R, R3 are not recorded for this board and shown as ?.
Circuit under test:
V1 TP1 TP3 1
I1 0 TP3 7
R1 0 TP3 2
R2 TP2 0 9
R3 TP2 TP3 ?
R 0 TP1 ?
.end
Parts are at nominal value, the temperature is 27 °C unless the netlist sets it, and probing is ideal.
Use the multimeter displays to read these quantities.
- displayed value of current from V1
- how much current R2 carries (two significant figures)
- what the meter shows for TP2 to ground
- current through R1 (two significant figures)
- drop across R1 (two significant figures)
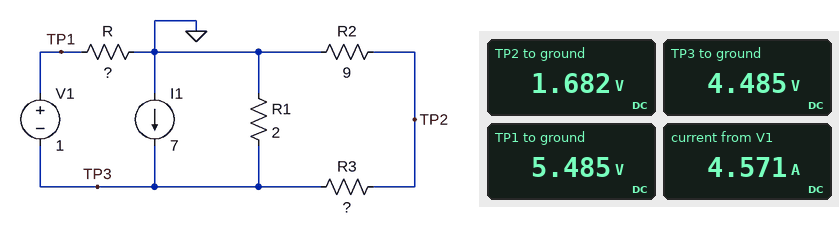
4.571 A
190 mA
1.682 V
2.2 A
4.5 V
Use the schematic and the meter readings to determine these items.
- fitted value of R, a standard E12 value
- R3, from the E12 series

1.2 Ω
15 Ω
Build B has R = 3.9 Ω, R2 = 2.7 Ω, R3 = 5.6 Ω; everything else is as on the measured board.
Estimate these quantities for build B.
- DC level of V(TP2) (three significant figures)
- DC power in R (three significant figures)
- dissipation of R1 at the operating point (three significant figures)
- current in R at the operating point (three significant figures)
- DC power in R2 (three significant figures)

2.50 V
19.4 W
29.6 W
2.23 A
2.32 W
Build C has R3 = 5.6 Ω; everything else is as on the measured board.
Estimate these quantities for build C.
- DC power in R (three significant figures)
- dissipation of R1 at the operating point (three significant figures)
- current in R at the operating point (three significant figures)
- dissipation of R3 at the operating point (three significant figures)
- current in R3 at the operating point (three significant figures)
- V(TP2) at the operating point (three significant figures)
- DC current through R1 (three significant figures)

24.3 W
9.68 W
4.50 A
508 mW
301 mA
2.71 V
2.20 A
